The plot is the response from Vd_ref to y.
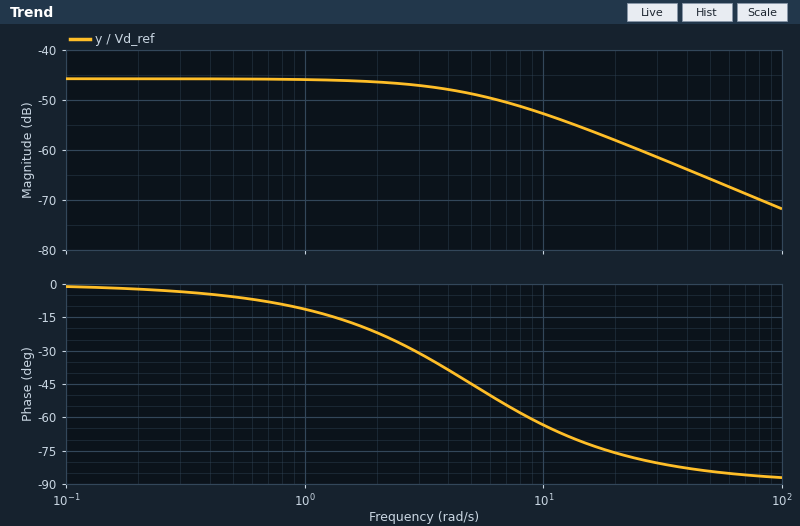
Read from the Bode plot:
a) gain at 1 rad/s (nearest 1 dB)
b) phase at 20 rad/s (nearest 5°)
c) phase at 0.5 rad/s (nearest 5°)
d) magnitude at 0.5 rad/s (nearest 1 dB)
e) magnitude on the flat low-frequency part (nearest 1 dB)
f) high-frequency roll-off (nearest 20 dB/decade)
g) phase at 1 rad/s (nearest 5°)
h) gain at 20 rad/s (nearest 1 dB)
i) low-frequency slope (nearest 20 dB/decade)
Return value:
-46 dB
-75°
-5°
-46 dB
-46 dB
-20 dB/decade
-10°
-58 dB
0 dB/decade
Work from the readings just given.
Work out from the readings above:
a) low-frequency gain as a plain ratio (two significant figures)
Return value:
0.0050
